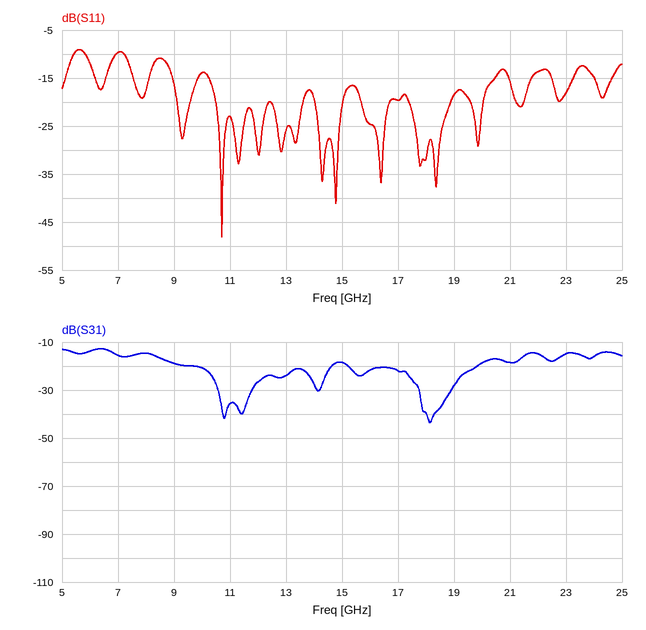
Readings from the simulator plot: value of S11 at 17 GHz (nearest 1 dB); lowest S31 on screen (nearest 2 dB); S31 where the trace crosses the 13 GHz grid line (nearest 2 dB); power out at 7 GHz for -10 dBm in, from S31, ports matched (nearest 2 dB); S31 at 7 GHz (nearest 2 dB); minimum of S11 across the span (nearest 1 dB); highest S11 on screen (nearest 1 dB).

-20 dB
-44 dB
-24 dB
-26 dBm
-16 dB
-48 dB
-9 dB
